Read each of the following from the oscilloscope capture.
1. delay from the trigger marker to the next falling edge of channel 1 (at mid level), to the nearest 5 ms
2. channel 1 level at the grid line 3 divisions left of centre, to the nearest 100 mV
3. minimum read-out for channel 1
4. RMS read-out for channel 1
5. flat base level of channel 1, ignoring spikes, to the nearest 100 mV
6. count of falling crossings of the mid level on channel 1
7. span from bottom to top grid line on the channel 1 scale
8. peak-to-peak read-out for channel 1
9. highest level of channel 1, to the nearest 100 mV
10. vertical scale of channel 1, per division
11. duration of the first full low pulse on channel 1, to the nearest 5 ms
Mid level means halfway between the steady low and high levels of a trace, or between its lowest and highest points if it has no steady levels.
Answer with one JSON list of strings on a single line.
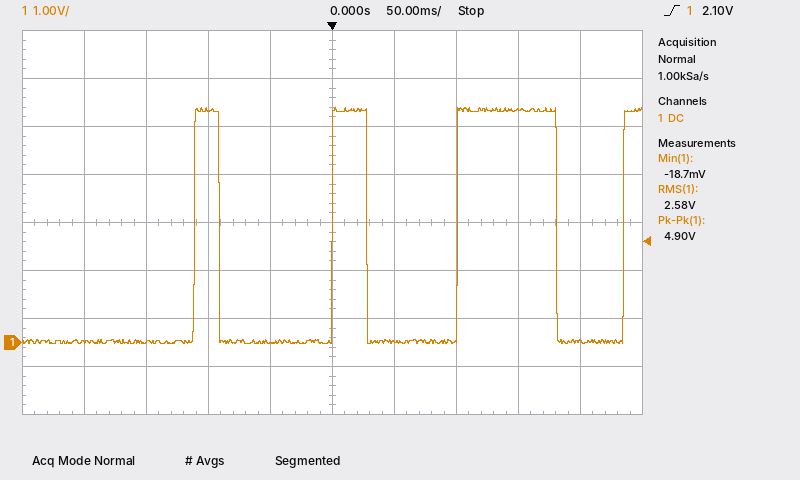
["30 ms", "0.0 V", "-18.7 mV", "2.58 V", "0.0 V", "3", "8 V", "4.90 V", "4.9 V", "1 V", "90 ms"]
